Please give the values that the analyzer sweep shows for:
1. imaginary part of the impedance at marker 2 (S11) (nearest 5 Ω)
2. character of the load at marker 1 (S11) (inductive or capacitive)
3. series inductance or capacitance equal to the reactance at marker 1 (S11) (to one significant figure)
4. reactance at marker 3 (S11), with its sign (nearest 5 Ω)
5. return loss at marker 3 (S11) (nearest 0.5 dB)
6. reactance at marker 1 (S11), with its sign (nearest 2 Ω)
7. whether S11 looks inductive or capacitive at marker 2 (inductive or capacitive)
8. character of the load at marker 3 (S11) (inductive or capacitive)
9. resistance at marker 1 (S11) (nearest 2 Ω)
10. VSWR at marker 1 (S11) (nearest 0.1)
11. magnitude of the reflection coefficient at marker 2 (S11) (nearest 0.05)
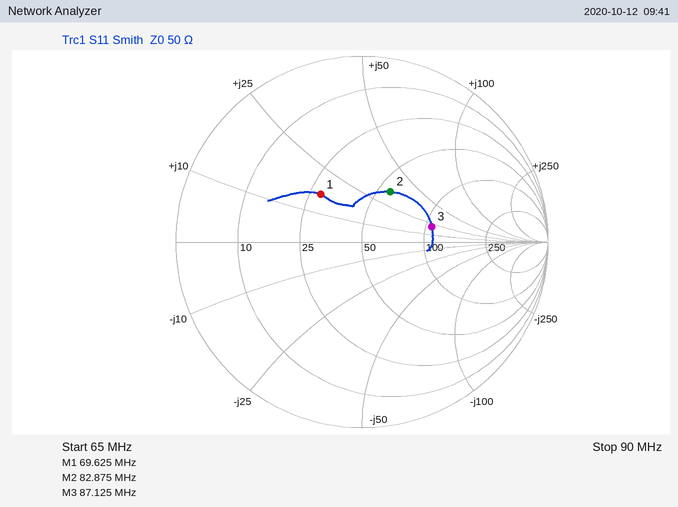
+35 Ω
inductive
40 nH
+20 Ω
8.5 dB
+16 Ω
inductive
inductive
28 Ω
2.0
0.30
